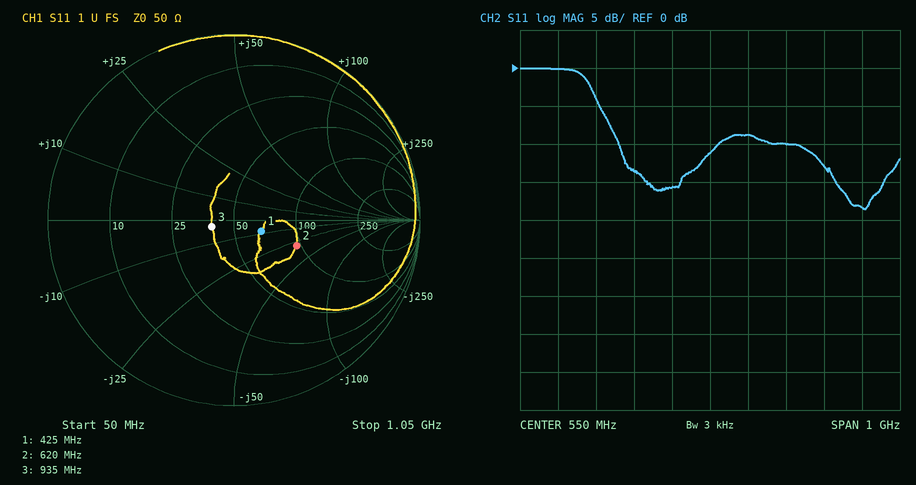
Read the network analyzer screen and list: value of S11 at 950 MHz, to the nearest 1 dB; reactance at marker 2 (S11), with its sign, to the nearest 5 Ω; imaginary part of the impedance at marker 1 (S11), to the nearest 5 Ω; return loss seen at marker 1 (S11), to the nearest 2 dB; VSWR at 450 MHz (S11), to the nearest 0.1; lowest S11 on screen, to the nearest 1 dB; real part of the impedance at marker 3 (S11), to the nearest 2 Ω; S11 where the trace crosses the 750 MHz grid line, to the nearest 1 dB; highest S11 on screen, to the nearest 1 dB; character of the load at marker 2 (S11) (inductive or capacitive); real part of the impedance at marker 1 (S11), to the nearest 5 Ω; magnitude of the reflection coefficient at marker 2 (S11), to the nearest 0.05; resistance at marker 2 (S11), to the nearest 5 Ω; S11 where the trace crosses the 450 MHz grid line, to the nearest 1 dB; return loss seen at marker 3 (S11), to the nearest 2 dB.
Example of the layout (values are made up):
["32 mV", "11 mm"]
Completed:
["-18 dB", "-30 Ω", "-10 Ω", "16 dB", "1.4", "-19 dB", "40 Ω", "-10 dB", "0 dB", "capacitive", "65 Ω", "0.35", "95 Ω", "-16 dB", "18 dB"]
